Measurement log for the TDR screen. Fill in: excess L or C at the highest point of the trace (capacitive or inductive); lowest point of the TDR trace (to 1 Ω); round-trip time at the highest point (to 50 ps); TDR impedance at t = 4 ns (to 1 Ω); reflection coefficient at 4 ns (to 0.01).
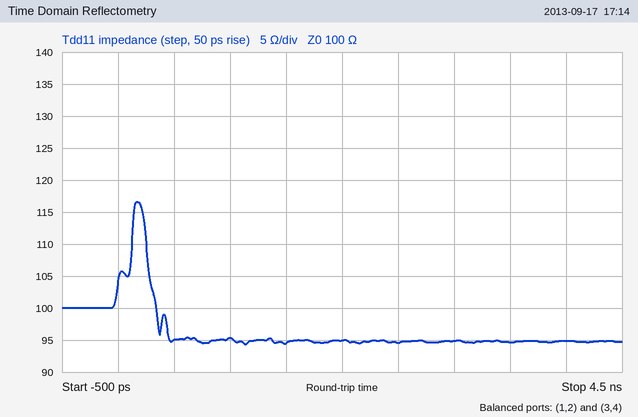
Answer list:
inductive
94 Ω
150 ps
95 Ω
-0.03
